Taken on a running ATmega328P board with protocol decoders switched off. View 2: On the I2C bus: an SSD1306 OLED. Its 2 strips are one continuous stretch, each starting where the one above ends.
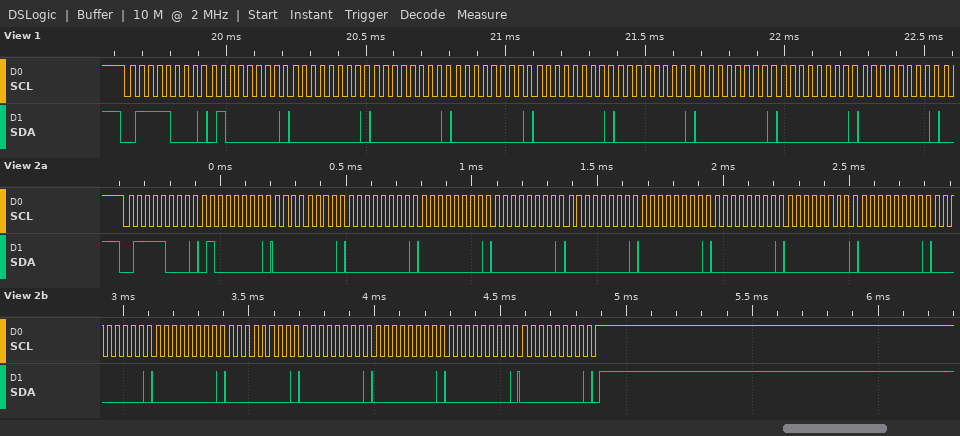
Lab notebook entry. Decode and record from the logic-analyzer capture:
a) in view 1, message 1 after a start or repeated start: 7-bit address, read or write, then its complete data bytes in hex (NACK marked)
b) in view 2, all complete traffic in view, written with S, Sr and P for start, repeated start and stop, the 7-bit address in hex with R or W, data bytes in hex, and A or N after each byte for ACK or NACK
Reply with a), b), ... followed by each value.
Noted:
a) 0x3C write: 40 00 00 00 00 00 00 00 00
b) S 3CW A 40 A 00 A 00 A 00 A 00 A 00 A 00 A 00 A 00 A 00 A 00 A 00 A 00 A 00 A 00 A 00 A 00 A P
